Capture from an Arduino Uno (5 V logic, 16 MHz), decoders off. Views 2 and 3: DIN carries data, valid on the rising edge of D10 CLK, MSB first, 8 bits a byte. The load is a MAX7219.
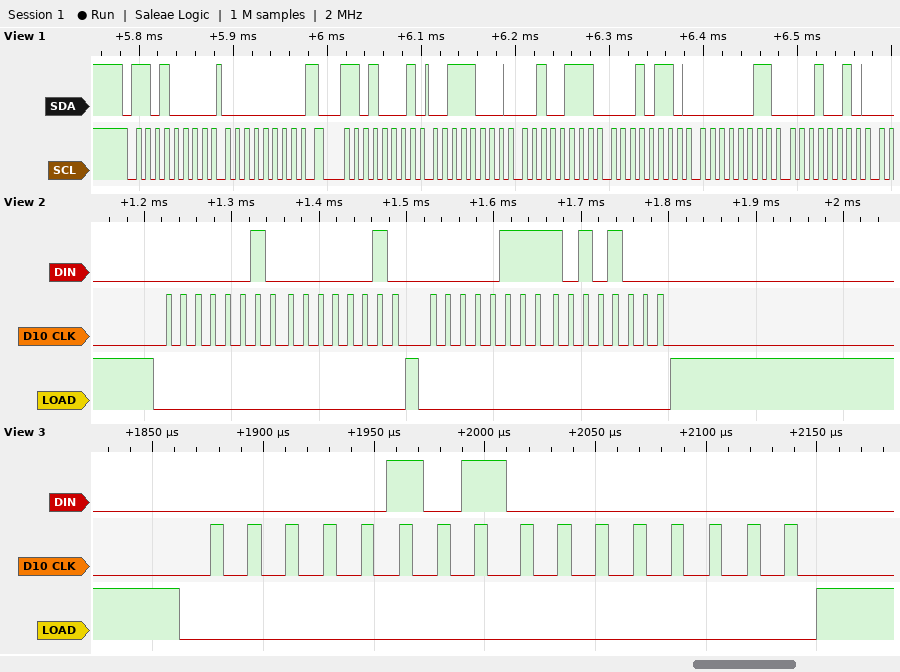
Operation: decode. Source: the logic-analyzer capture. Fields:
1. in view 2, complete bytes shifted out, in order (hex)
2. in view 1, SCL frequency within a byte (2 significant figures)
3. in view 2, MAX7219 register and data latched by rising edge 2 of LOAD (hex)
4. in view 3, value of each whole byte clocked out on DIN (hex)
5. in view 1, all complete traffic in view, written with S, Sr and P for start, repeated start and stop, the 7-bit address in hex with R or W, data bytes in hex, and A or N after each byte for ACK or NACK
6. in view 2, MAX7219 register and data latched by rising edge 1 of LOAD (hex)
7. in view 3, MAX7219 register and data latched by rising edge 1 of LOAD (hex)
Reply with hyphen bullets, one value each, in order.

- 0x02 0x02 0x07 0xA8
- 100 kHz
- register 0x7, data 0xA8
- 0x05 0x00
- S 68W A 00 A Sr 68R A 38 A 27 A 16 A 03 A 12 A
- register 0x2, data 0x02
- register 0x5, data 0x00
